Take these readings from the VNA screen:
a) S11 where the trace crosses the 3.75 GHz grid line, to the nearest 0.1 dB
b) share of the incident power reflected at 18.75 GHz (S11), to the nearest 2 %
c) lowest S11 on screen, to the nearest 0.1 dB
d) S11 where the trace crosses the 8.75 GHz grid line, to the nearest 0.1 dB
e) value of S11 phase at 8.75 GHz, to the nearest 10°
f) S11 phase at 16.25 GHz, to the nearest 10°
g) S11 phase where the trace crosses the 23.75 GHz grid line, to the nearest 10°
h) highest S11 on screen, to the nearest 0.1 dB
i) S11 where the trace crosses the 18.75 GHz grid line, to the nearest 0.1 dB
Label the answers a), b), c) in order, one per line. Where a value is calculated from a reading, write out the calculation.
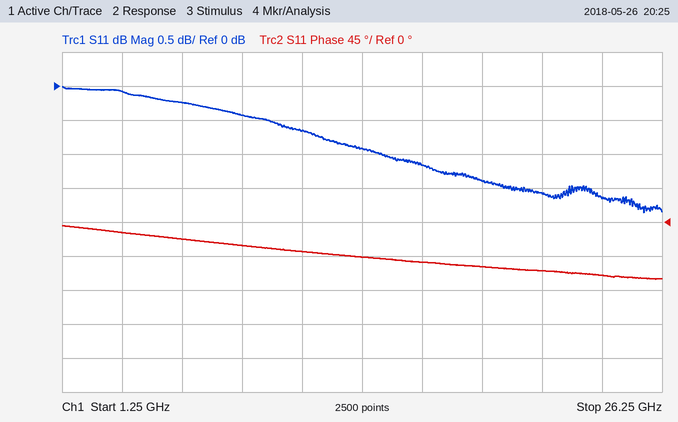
a) -0.1 dB
b) 10^(-1.4/10) ≈ 72 %
c) -1.9 dB
d) -0.4 dB
e) -30°
f) -50°
g) -70°
h) 0.0 dB
i) -1.4 dB
